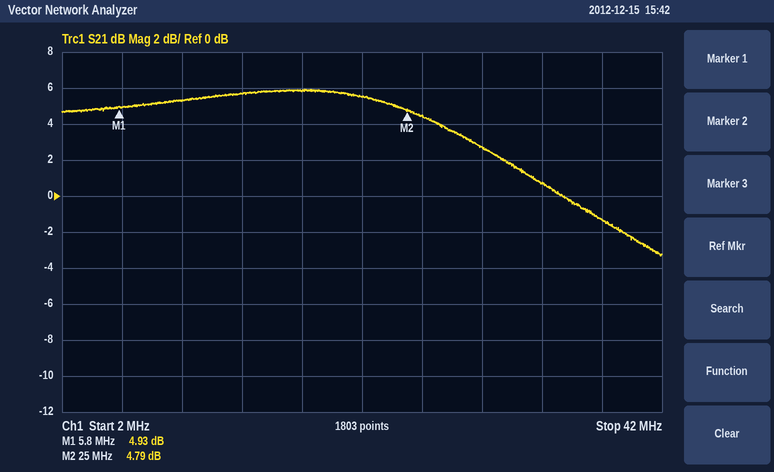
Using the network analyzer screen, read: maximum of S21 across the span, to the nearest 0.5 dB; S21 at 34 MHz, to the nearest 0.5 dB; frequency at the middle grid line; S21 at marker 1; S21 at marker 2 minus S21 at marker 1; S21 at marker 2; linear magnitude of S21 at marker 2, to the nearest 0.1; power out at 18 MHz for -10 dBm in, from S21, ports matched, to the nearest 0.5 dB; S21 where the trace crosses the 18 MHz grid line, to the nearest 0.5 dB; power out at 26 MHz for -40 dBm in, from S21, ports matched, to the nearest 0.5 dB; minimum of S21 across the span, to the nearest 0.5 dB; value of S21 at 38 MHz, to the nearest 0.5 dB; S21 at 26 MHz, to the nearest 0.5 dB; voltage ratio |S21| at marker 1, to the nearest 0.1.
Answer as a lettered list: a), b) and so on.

a) 6.0 dB
b) 0.5 dB
c) 22 MHz
d) 4.93 dB
e) -0.14 dB
f) 4.79 dB
g) 1.7
h) -4.0 dBm
i) 6.0 dB
j) -35.5 dBm
k) -3.5 dB
l) -1.5 dB
m) 4.5 dB
n) 1.8
